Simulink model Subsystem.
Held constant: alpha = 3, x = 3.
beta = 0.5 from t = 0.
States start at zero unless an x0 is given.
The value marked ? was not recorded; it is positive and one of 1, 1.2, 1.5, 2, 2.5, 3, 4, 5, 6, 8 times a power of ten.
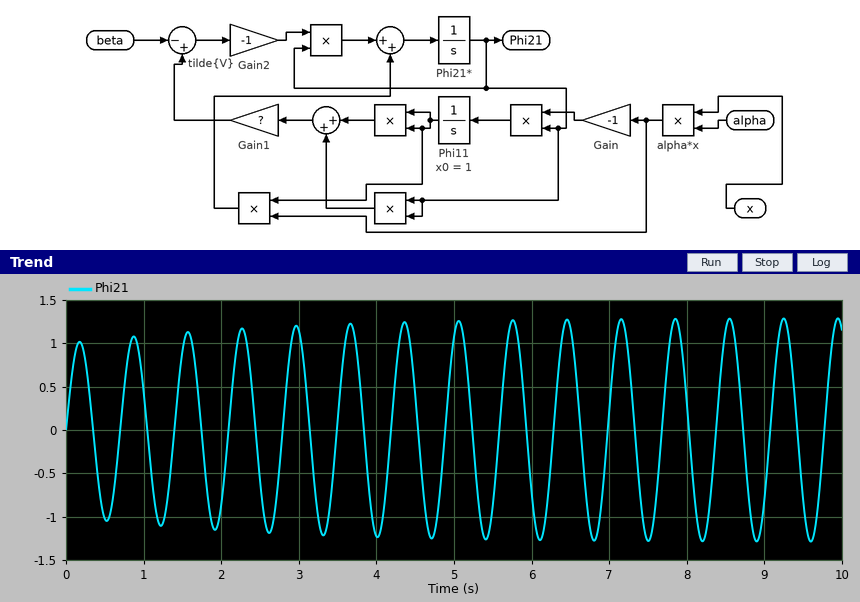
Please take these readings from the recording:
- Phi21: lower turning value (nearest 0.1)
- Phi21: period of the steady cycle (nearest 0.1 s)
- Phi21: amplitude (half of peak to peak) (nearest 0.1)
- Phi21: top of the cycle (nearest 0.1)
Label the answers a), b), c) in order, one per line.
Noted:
a) -1.3
b) 0.7 s
c) 1.3
d) 1.3
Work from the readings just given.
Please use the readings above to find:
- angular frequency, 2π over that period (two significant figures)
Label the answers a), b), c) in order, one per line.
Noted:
a) 9.0 rad/s
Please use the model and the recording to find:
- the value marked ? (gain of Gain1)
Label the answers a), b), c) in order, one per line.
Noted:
a) 0.3
